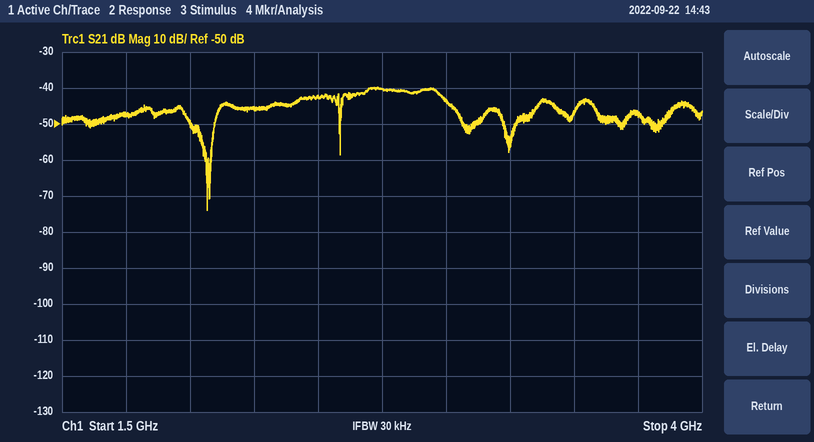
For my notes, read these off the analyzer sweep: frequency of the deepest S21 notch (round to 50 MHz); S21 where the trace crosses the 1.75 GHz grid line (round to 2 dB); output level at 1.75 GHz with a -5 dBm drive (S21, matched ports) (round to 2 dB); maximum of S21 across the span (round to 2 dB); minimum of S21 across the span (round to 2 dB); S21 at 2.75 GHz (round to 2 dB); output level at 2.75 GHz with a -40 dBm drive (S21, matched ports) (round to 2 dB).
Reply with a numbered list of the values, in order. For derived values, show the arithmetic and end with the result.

1. 2.05 GHz
2. -48 dB
3. -5 dBm + (-48 dB) = -52 dBm
4. -40 dB
5. -74 dB
6. -40 dB
7. -40 dBm + (-40 dB) = -80 dBm
